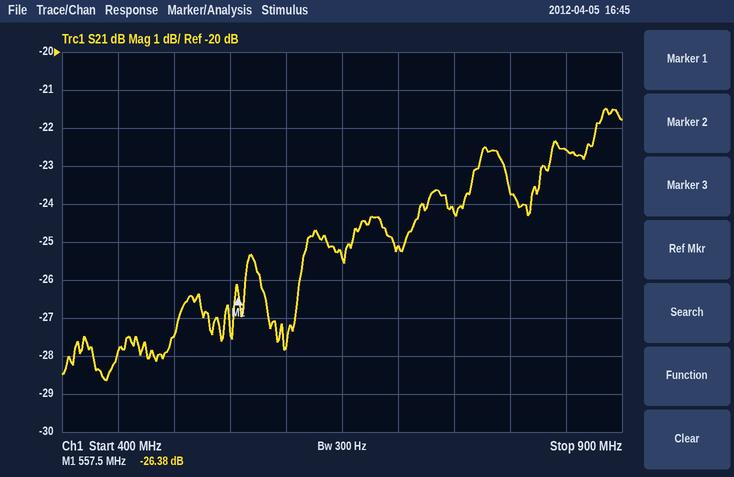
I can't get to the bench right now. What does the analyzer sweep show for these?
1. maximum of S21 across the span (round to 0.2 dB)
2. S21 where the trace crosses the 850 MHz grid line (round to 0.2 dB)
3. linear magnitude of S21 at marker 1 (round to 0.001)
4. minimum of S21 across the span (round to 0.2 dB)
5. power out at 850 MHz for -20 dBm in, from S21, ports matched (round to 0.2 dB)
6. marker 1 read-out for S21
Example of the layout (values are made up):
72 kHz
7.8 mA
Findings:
-21.4 dB
-22.6 dB
0.048
-28.6 dB
-42.6 dBm
-26.38 dB
